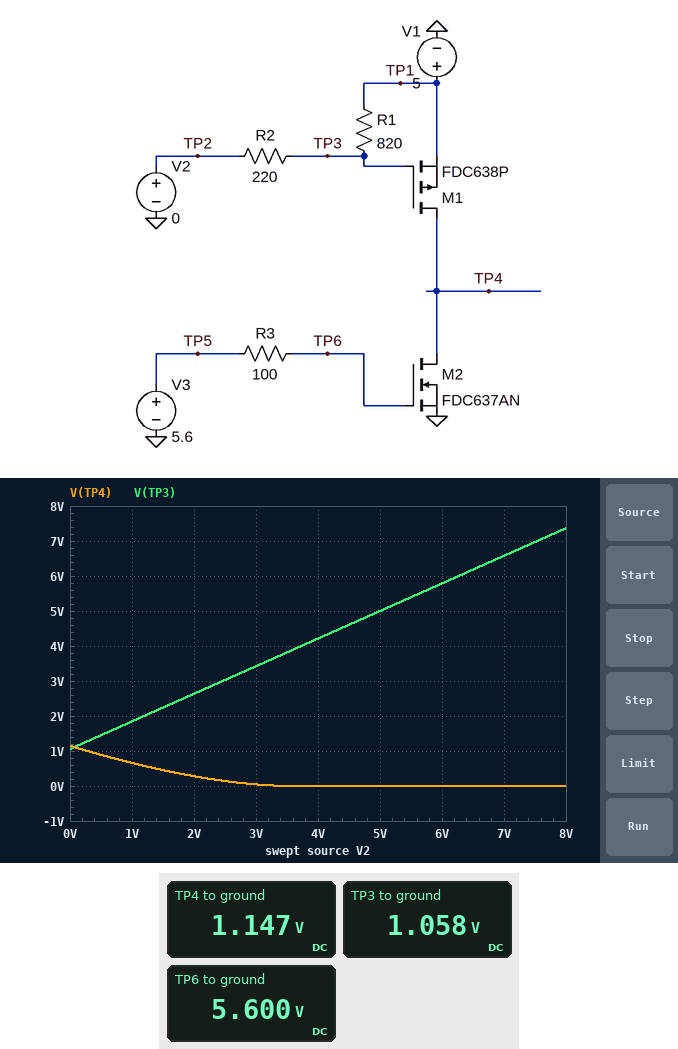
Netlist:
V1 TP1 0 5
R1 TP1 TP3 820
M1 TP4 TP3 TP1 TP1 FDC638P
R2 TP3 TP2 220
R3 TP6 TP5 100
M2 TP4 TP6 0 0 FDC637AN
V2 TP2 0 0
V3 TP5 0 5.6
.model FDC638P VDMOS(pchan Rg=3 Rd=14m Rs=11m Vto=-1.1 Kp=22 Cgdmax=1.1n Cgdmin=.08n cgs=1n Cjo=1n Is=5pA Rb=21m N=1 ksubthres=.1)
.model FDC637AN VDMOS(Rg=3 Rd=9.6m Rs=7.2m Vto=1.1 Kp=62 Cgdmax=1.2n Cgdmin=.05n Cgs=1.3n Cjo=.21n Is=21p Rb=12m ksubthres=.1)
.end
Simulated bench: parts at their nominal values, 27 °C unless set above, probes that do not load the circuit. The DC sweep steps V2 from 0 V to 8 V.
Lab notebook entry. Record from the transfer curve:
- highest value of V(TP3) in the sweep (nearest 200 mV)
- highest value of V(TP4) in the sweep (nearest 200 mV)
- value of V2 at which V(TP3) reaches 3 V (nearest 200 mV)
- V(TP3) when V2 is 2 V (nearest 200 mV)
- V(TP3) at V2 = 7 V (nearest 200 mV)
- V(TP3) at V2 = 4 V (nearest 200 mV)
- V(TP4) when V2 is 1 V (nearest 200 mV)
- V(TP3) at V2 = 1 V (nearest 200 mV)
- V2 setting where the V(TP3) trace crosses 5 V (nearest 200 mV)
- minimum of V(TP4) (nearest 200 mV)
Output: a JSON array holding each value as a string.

["7.4 V", "1.2 V", "2.4 V", "2.6 V", "6.6 V", "4.2 V", "600 mV", "1.8 V", "5.0 V", "0 V"]
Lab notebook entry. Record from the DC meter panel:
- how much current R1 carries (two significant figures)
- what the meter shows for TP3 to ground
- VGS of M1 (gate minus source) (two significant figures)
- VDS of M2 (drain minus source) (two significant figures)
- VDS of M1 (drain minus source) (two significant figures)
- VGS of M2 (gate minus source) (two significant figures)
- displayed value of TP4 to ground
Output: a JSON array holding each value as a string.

["4.8 mA", "1.058 V", "-3.9 V", "1.1 V", "-3.9 V", "5.6 V", "1.147 V"]
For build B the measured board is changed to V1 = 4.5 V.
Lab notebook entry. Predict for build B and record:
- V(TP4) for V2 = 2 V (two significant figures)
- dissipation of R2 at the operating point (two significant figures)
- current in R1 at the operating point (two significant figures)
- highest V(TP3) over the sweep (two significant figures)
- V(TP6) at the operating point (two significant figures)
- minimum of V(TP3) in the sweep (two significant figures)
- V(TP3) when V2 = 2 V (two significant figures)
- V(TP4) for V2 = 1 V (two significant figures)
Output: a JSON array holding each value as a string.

["140 mV", "4.1 mW", "4.3 mA", "7.3 V", "5.6 V", "950 mV", "2.5 V", "450 mV"]
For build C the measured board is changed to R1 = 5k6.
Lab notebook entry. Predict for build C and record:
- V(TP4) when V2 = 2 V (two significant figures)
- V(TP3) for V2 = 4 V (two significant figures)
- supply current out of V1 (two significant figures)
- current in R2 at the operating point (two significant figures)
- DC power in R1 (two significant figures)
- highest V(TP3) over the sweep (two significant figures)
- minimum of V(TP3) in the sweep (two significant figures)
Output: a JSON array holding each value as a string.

["520 mV", "4.0 V", "74 A", "860 µA", "4.1 mW", "7.9 V", "190 mV"]
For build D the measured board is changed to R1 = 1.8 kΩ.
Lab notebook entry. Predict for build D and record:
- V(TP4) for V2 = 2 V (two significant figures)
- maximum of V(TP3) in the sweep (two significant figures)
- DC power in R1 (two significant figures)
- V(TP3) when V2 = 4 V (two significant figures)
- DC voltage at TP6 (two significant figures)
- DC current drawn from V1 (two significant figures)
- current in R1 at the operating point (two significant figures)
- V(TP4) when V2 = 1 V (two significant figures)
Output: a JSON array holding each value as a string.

["410 mV", "7.7 V", "11 mW", "4.1 V", "5.6 V", "68 A", "2.5 mA", "900 mV"]
